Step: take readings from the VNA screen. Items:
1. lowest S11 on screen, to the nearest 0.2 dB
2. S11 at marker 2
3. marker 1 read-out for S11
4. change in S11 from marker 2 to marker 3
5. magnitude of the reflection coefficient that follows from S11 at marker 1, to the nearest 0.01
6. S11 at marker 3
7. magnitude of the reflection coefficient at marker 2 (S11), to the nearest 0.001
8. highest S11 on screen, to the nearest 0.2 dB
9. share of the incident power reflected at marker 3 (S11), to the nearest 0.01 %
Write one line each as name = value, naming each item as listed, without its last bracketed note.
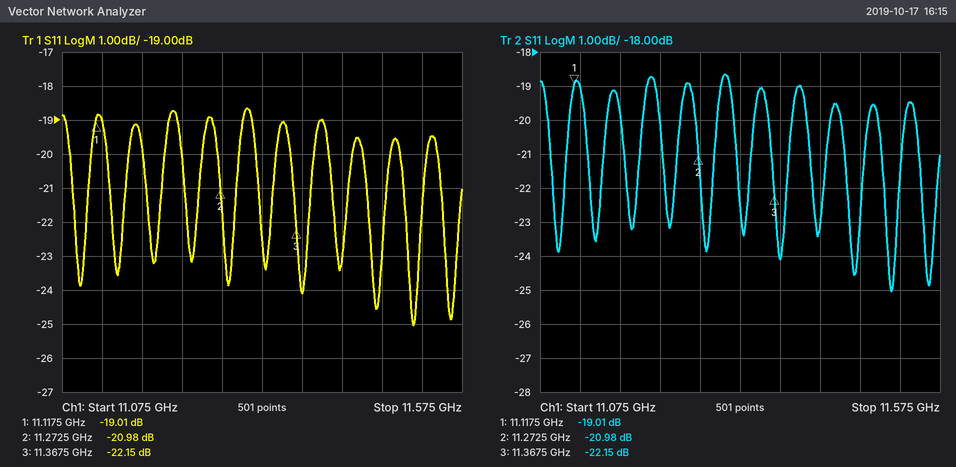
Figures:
lowest S11 on screen, to the nearest 0.2 dB = -25.0 dB
S11 at marker 2 = -20.98 dB
marker 1 read-out for S11 = -19.01 dB
change in S11 from marker 2 to marker 3 = -1.17 dB
magnitude of the reflection coefficient that follows from S11 at marker 1, to the nearest 0.01 = 0.11
S11 at marker 3 = -22.15 dB
magnitude of the reflection coefficient at marker 2 (S11), to the nearest 0.001 = 0.089
highest S11 on screen, to the nearest 0.2 dB = -18.6 dB
share of the incident power reflected at marker 3 (S11), to the nearest 0.01 % = 0.61 %
